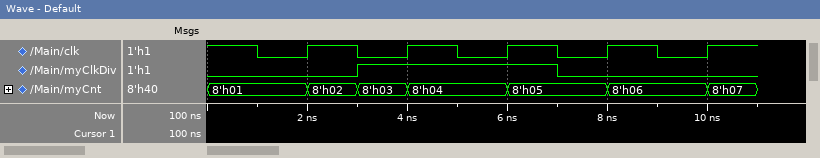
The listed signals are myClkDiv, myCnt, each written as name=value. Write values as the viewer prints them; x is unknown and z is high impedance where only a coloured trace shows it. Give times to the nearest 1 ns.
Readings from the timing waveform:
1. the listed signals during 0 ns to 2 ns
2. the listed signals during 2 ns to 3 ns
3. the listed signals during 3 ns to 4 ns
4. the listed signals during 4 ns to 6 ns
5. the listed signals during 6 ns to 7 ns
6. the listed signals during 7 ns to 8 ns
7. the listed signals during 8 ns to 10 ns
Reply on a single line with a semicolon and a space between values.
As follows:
myClkDiv=0, myCnt=8'h01; myClkDiv=0, myCnt=8'h02; myClkDiv=1, myCnt=8'h03; myClkDiv=1, myCnt=8'h04; myClkDiv=1, myCnt=8'h05; myClkDiv=0, myCnt=8'h05; myClkDiv=0, myCnt=8'h06
